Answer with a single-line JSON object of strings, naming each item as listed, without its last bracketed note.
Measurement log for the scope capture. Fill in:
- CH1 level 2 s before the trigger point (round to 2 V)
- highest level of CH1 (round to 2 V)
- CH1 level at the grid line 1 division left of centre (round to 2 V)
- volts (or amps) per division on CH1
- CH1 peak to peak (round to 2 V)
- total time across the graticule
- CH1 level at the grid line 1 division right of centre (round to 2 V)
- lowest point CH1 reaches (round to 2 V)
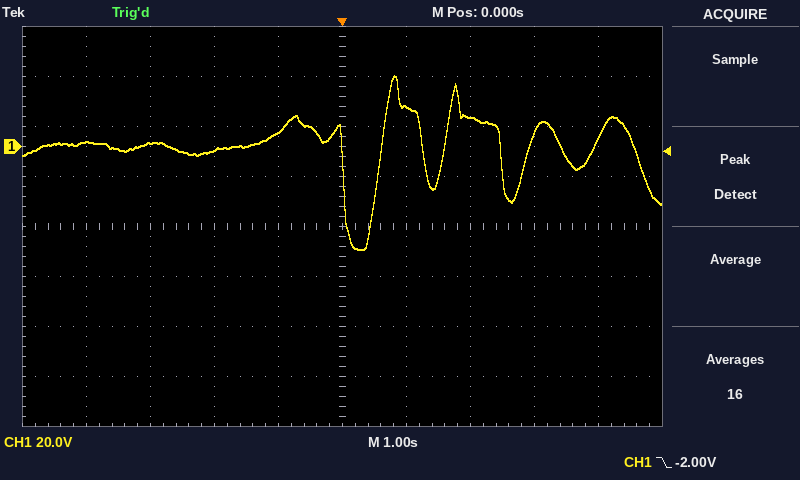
{"CH1 level 2 s before the trigger point": "-2 V", "highest level of CH1": "28 V", "CH1 level at the grid line 1 division left of centre": "6 V", "volts (or amps) per division on CH1": "20 V", "CH1 peak to peak": "70 V", "total time across the graticule": "10 s", "CH1 level at the grid line 1 division right of centre": "16 V", "lowest point CH1 reaches": "-42 V"}
